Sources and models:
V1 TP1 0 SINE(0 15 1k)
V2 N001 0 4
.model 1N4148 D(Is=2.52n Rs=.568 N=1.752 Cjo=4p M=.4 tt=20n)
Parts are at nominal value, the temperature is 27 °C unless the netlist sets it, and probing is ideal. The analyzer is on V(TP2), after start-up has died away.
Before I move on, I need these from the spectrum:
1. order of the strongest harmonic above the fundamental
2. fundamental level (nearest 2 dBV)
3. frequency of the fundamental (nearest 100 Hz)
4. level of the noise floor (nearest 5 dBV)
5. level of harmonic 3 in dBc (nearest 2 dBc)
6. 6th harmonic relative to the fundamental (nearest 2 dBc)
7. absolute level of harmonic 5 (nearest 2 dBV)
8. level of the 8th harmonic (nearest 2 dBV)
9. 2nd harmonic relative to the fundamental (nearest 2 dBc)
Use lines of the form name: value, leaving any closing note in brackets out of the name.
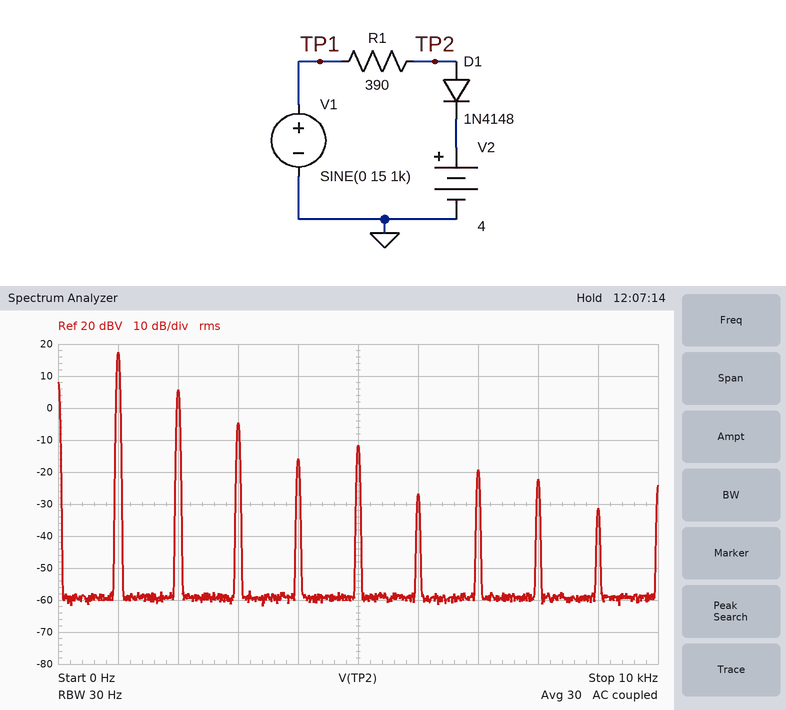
order of the strongest harmonic above the fundamental: 2
fundamental level: 18 dBV
frequency of the fundamental: 1.0 kHz
level of the noise floor: -60 dBV
level of harmonic 3 in dBc: -22 dBc
6th harmonic relative to the fundamental: -44 dBc
absolute level of harmonic 5: -12 dBV
level of the 8th harmonic: -22 dBV
2nd harmonic relative to the fundamental: -12 dBc
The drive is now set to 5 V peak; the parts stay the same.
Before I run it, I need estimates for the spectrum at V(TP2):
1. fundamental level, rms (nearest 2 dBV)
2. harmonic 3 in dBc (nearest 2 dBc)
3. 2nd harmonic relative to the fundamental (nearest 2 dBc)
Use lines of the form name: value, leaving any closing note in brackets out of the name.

fundamental level, rms: 10 dBV
harmonic 3 in dBc: -38 dBc
2nd harmonic relative to the fundamental: -36 dBc
